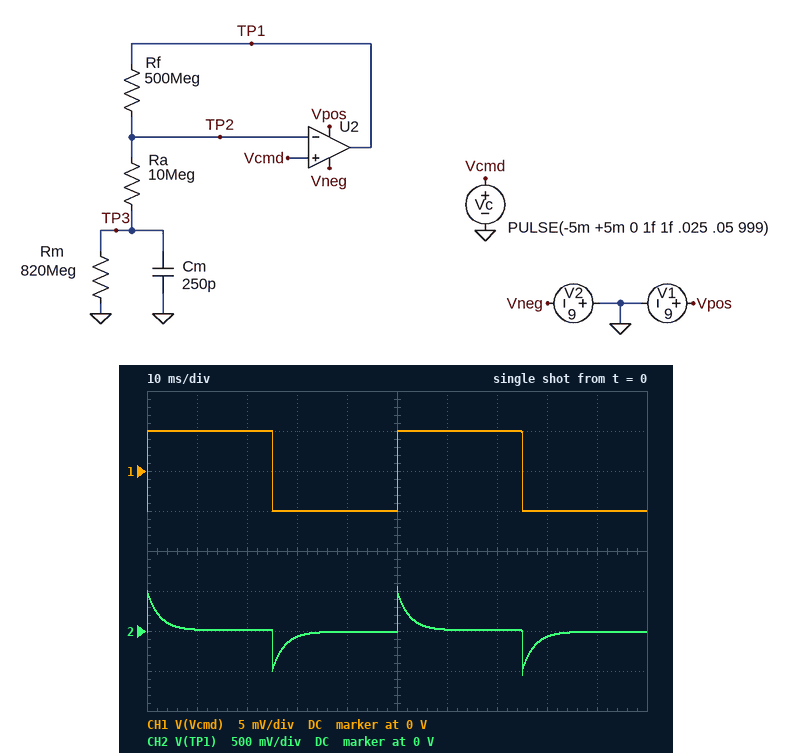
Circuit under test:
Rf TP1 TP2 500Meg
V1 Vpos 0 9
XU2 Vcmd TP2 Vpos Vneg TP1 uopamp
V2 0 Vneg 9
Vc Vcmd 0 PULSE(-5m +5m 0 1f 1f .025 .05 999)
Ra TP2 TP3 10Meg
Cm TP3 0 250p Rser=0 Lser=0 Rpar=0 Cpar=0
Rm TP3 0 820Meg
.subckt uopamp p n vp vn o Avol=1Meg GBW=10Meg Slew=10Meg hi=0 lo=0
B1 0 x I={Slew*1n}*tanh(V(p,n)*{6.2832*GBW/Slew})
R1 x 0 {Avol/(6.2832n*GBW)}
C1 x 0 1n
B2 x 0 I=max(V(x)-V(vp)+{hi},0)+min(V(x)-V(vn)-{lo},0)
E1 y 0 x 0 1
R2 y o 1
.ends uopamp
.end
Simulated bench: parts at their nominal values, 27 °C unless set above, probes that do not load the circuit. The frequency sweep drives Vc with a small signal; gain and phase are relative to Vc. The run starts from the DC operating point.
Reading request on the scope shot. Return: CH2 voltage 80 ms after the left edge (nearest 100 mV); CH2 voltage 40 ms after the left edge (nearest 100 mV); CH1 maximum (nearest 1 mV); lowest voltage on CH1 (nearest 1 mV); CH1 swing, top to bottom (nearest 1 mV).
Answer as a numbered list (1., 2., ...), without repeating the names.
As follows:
1. -100 mV
2. 0 V
3. 5 mV
4. -5 mV
5. 10 mV
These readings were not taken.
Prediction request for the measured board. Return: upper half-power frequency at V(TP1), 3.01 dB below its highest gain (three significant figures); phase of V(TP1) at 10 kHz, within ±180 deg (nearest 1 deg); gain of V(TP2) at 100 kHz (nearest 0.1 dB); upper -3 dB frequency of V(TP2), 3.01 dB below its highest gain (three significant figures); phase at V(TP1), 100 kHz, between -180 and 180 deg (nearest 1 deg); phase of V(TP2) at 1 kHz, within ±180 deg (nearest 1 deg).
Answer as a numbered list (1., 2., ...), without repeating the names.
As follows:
1. 196 kHz
2. -3 deg
3. -1.0 dB
4. 196 kHz
5. -27 deg
6. 0 deg
